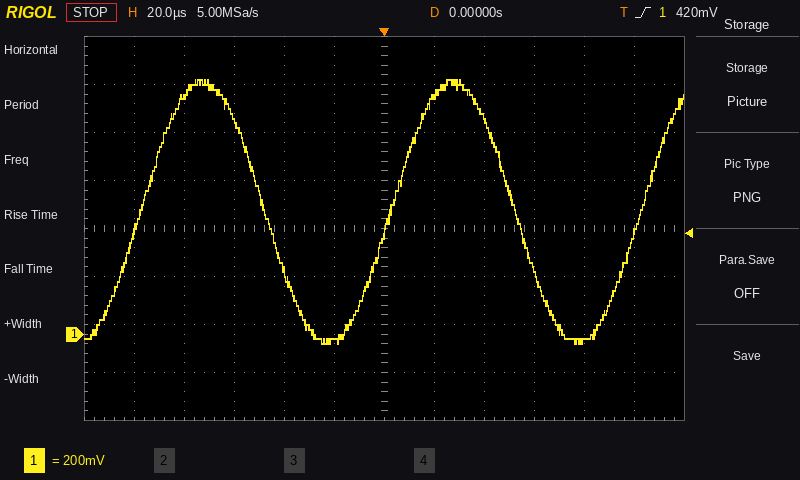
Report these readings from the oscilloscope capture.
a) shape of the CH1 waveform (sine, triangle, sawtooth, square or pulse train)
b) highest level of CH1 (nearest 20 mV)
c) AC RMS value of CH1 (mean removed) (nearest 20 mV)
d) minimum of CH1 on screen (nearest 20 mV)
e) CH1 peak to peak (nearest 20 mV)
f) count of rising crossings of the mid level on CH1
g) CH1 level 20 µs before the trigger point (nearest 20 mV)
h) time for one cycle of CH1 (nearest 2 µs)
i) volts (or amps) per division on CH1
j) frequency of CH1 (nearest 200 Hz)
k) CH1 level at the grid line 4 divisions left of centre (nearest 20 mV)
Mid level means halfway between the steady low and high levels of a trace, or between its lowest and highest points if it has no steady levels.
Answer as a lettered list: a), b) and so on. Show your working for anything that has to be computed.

a) sine
b) 1.06 V
c) 1.10 V / (2√2) ≈ 389 mV, so 380 mV to the nearest 20 mV
d) -40 mV
e) 1.06 V − (-40 mV) = 1.10 V
f) 3
g) -20 mV
h) 100 µs
i) 200 mV
j) 1 / 100 µs ≈ 10.0 kHz
k) 1.00 V
